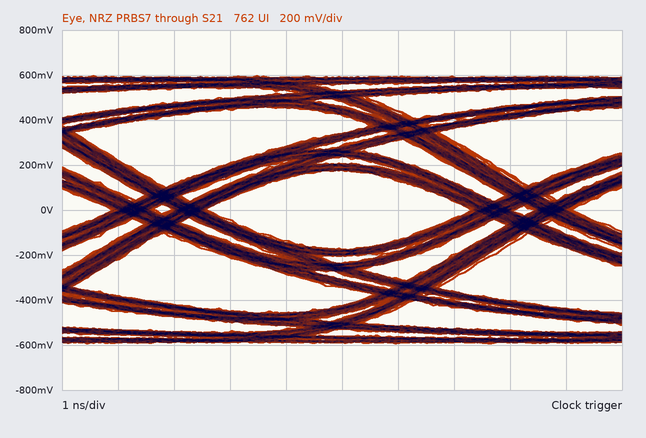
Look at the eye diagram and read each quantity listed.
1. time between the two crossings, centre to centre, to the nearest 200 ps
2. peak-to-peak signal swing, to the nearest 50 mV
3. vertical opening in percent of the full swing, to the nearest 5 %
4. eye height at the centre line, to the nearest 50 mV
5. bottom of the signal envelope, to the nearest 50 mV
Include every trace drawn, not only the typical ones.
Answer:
6.4 ns
1.20 V
30 %
350 mV
-600 mV
